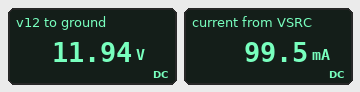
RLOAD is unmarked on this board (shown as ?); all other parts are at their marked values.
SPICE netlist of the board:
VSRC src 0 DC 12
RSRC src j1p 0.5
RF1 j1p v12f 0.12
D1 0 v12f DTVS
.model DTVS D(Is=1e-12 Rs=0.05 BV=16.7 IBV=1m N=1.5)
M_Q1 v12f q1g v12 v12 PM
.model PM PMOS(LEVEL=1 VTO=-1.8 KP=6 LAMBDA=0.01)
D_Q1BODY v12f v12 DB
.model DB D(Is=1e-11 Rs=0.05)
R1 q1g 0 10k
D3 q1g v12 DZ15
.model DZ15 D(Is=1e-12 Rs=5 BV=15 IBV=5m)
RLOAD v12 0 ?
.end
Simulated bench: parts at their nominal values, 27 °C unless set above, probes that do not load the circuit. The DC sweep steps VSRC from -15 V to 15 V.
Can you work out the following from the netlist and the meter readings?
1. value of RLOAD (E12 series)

120 Ω
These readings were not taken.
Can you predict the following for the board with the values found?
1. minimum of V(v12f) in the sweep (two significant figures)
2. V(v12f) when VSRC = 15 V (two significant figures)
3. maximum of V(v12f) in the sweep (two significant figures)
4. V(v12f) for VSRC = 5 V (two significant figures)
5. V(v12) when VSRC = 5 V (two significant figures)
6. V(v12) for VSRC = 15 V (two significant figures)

-2.2 V
15 V
15 V
5.0 V
5.0 V
15 V
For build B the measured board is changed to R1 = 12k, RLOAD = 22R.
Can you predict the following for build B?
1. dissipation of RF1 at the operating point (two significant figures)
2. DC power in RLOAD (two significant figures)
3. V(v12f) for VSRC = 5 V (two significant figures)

34 mW
6.2 W
4.9 V
